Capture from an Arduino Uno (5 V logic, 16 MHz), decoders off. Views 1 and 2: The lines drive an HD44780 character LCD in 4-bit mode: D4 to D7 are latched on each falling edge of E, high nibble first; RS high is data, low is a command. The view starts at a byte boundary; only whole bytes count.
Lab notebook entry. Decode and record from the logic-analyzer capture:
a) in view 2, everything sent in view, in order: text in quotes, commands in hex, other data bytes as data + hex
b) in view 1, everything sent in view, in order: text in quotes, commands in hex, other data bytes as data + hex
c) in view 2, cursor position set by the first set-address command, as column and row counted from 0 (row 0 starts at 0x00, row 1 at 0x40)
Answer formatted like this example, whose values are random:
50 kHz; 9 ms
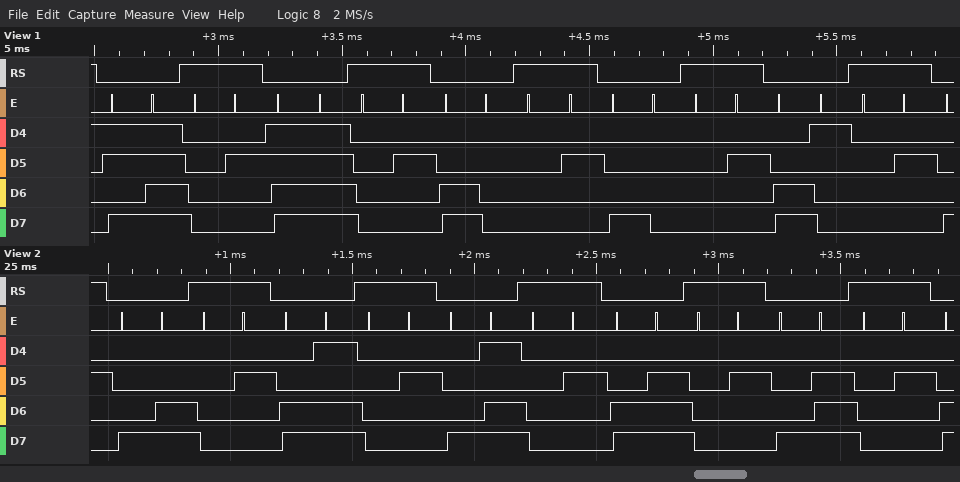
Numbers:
0x8C data 02 0xCD data 02 0x8D data 02 0xCE data 02 0x8E data 02; 0xBF data 02 0xFF data 02 0xC0 data 02 0x80 data 02 0xC1 data 02; column 12, row 0
